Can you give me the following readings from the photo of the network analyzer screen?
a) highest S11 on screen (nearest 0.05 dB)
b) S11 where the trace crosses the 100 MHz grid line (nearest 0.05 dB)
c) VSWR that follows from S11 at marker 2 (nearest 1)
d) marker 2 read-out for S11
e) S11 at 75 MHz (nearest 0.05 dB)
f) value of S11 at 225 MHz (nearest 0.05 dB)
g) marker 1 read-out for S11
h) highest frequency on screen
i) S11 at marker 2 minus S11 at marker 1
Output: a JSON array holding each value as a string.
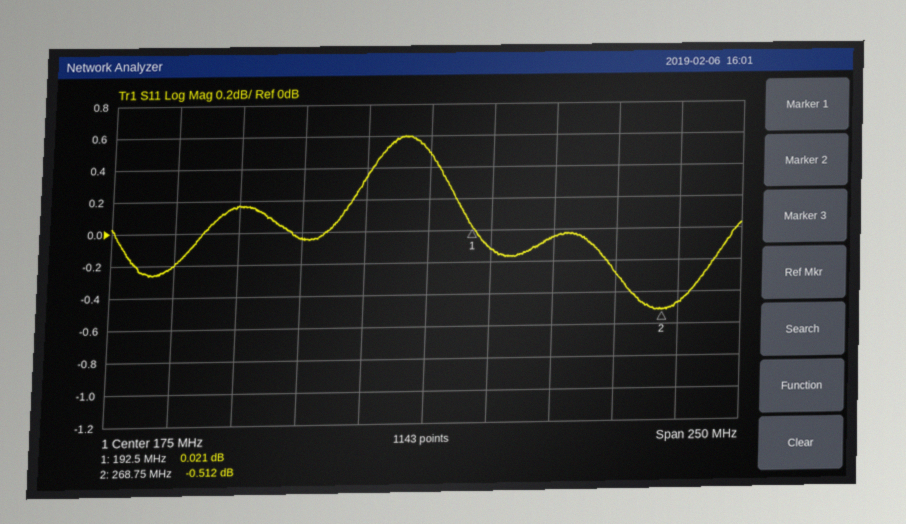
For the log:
["0.60 dB", "0.15 dB", "34", "-0.512 dB", "-0.20 dB", "-0.05 dB", "0.021 dB", "300 MHz", "-0.533 dB"]
